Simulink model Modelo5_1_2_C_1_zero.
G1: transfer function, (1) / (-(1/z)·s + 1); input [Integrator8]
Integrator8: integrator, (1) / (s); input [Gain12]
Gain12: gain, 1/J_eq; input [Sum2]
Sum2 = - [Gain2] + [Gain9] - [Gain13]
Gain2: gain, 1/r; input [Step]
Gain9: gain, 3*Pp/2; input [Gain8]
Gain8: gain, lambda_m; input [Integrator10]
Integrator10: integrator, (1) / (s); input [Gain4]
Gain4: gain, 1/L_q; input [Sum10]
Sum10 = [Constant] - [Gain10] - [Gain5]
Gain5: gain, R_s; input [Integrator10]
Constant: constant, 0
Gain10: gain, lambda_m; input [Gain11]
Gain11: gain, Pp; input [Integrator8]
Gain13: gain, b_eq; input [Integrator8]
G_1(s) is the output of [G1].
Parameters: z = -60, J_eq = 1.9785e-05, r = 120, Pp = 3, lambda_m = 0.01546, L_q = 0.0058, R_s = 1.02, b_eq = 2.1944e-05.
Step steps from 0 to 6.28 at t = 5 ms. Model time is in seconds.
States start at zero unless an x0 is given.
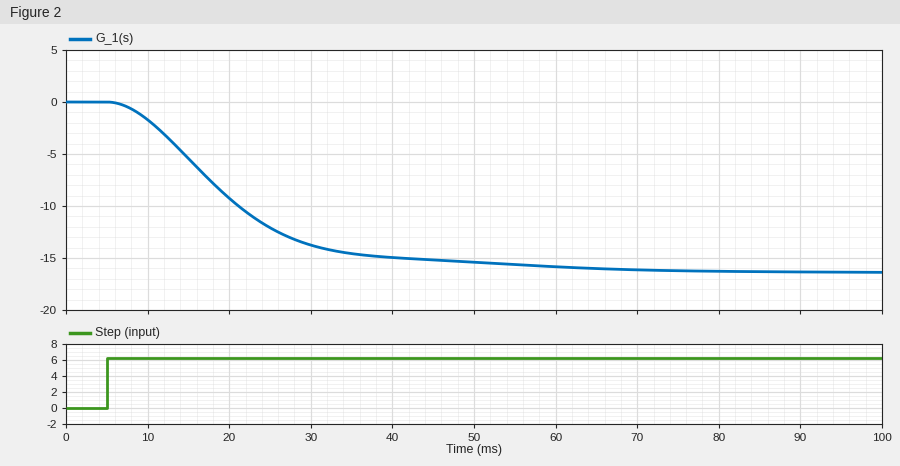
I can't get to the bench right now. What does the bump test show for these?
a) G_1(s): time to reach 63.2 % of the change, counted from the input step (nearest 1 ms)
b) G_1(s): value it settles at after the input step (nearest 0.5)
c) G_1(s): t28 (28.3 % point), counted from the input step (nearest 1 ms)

17 ms
-16.5
9 ms
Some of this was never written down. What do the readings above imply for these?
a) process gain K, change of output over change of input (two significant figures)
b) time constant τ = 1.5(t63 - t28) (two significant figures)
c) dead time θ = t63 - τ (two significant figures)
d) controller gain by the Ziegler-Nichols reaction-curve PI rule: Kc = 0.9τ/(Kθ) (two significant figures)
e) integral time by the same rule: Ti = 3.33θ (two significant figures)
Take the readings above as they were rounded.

-2.6
12 ms
5.0 ms
-0.83
17 ms
